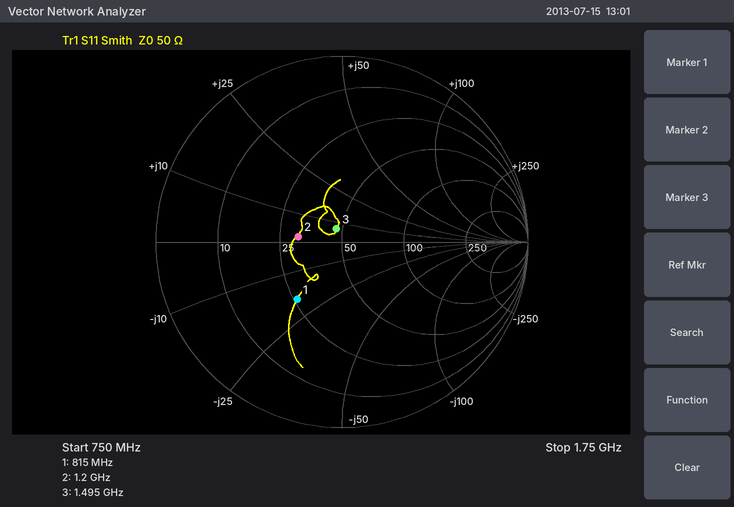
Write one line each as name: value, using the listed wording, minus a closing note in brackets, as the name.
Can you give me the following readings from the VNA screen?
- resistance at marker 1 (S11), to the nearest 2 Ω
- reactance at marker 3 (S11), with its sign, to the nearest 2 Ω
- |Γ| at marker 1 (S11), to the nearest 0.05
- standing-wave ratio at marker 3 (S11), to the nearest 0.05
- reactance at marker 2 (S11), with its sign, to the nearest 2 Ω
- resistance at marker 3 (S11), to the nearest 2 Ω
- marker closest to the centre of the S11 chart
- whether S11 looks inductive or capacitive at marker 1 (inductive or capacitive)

resistance at marker 1 (S11), to the nearest 2 Ω: 26 Ω
reactance at marker 3 (S11), with its sign, to the nearest 2 Ω: +6 Ω
|Γ| at marker 1 (S11), to the nearest 0.05: 0.40
standing-wave ratio at marker 3 (S11), to the nearest 0.05: 1.15
reactance at marker 2 (S11), with its sign, to the nearest 2 Ω: +2 Ω
resistance at marker 3 (S11), to the nearest 2 Ω: 46 Ω
marker closest to the centre of the S11 chart: marker 3
whether S11 looks inductive or capacitive at marker 1: capacitive
